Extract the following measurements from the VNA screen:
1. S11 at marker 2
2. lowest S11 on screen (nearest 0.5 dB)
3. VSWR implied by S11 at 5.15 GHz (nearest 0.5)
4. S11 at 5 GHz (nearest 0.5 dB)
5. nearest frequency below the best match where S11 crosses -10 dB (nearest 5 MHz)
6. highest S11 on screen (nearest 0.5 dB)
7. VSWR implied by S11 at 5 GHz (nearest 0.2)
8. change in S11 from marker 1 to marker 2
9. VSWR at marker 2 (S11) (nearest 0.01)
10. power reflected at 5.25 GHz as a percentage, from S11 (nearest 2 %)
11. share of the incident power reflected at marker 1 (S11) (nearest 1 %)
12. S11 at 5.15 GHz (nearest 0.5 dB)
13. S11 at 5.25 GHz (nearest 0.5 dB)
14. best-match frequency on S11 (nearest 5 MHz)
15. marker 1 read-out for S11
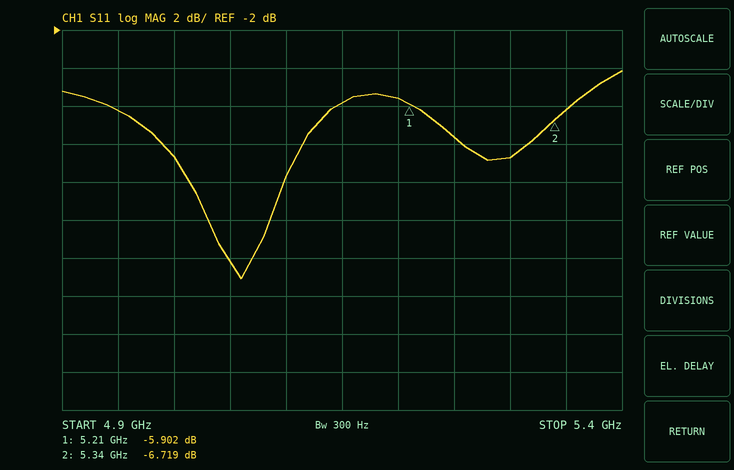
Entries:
-6.719 dB
-15.0 dB
3.0
-8.5 dB
5.015 GHz
-4.0 dB
2.2
-0.817 dB
2.71
18 %
26 %
-6.0 dB
-7.5 dB
5.060 GHz
-5.902 dB
